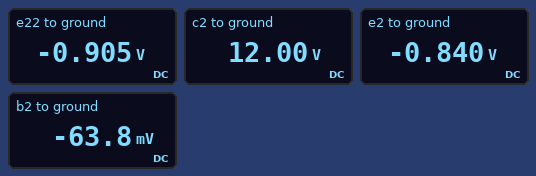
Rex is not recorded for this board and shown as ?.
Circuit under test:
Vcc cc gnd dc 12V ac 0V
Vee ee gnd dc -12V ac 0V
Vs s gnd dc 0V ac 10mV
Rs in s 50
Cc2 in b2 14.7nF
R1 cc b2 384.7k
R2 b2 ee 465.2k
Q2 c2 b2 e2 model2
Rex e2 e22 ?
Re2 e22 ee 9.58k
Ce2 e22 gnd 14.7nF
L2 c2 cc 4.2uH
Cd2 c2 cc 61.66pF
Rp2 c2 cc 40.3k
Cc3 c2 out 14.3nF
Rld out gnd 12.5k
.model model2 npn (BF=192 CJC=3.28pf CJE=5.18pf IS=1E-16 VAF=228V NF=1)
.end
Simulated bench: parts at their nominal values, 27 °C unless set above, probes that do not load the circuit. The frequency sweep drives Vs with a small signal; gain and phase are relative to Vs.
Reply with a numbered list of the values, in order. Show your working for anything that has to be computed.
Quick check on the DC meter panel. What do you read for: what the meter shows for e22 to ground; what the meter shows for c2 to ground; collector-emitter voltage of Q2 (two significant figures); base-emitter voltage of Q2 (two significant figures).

1. -0.905 V
2. 12.00 V
3. 12 V - (-840 mV) = 13 V
4. -63.8 mV - (-840 mV) = 780 mV
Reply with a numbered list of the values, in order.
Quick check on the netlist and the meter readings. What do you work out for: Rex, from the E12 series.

1. 56 Ω
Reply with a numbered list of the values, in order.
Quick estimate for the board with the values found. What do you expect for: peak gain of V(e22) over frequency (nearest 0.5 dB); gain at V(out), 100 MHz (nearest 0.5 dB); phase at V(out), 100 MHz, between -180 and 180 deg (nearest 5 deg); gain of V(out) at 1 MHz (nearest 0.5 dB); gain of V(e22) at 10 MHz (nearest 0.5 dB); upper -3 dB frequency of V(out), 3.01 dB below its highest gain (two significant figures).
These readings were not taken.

1. 0 dB
2. -10.0 dB
3. 75 deg
4. -9.5 dB
5. -39.0 dB
6. 9.9 MHz
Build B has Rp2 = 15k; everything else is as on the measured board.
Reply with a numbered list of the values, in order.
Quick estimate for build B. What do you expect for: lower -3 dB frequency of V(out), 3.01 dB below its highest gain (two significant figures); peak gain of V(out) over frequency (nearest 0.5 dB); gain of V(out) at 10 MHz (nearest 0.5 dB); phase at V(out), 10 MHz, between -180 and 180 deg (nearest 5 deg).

1. 9.5 MHz
2. 38.5 dB
3. 33.5 dB
4. 125 deg
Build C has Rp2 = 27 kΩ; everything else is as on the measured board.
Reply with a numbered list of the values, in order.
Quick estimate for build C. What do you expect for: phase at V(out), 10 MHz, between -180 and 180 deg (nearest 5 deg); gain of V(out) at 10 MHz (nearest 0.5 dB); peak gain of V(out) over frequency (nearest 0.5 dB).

1. 120 deg
2. 34.0 dB
3. 40.5 dB
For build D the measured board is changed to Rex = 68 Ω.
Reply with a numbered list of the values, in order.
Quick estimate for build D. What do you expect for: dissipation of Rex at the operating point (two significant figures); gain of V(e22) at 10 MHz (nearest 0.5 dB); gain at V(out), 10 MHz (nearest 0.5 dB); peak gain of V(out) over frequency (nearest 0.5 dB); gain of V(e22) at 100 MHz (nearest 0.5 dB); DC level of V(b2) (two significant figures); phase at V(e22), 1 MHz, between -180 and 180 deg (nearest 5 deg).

1. 91 µW
2. -40.0 dB
3. 33.5 dB
4. 40.0 dB
5. -58.5 dB
6. -62 mV
7. -85 deg
